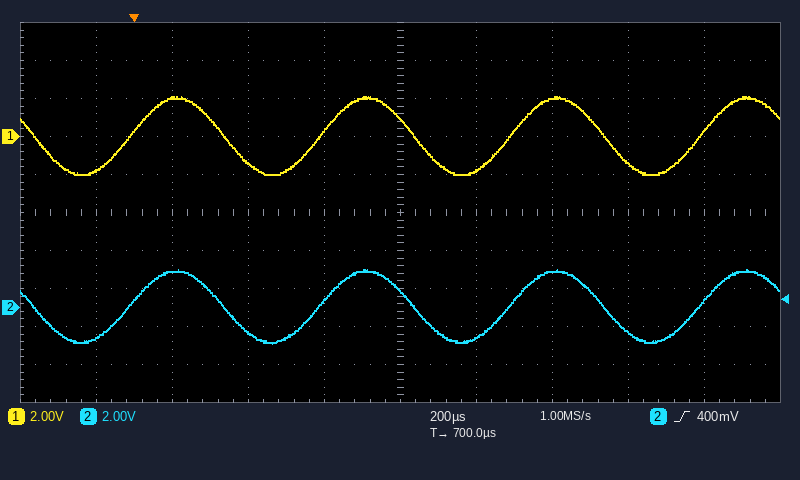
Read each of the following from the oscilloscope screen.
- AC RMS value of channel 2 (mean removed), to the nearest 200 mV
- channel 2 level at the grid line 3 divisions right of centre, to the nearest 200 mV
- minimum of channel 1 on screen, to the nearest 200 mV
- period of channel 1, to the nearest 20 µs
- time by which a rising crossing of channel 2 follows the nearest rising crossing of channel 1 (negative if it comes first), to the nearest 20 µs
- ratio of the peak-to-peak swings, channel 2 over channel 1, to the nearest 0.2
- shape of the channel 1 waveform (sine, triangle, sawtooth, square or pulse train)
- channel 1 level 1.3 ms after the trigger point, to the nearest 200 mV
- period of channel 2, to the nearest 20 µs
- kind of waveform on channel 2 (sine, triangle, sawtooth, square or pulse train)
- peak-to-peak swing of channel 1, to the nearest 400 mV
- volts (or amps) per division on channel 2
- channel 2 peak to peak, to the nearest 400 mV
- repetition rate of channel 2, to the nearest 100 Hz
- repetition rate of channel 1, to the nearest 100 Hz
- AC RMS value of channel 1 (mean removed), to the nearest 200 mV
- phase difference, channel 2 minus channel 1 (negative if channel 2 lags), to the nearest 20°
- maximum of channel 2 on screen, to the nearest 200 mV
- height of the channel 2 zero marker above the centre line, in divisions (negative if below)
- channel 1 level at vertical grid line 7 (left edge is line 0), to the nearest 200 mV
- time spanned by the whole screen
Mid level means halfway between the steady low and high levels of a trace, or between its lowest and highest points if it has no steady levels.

1.4 V
-1.2 V
-2.0 V
500 µs
0 µs
1.0
sine
-1.4 V
500 µs
sine
4.0 V
2 V
4.0 V
2.0 kHz
2.0 kHz
1.4 V
0°
2.0 V
-2.5 div
2.0 V
2 ms
